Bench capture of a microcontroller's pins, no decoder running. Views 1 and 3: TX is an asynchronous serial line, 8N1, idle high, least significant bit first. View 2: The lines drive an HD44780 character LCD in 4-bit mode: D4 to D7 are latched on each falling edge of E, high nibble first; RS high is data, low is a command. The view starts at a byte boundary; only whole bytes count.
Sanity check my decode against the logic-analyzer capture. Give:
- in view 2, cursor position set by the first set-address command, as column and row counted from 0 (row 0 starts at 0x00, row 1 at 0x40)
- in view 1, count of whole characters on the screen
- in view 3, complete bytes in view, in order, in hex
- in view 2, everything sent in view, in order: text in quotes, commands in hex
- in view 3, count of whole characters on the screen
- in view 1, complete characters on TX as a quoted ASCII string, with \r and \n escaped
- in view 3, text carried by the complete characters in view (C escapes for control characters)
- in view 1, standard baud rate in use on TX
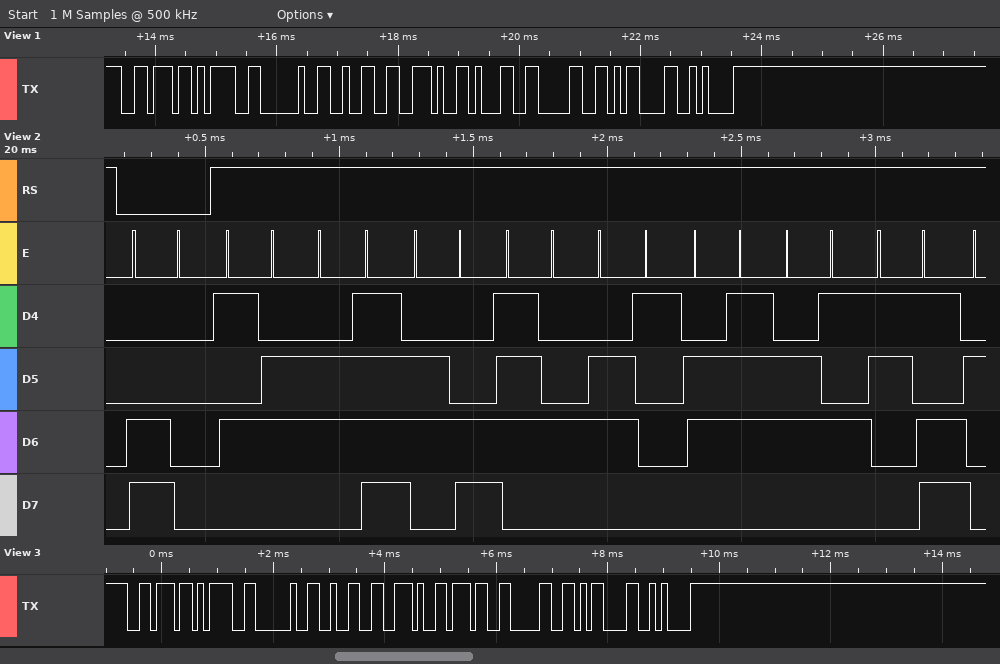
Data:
column 0, row 1
9
76 3D 20 32 2E 37 30 0D 0A
0xC0 "Voltage="
9
"v= 2.10\r\n"
"v= 2.70\r\n"
9600 baud
